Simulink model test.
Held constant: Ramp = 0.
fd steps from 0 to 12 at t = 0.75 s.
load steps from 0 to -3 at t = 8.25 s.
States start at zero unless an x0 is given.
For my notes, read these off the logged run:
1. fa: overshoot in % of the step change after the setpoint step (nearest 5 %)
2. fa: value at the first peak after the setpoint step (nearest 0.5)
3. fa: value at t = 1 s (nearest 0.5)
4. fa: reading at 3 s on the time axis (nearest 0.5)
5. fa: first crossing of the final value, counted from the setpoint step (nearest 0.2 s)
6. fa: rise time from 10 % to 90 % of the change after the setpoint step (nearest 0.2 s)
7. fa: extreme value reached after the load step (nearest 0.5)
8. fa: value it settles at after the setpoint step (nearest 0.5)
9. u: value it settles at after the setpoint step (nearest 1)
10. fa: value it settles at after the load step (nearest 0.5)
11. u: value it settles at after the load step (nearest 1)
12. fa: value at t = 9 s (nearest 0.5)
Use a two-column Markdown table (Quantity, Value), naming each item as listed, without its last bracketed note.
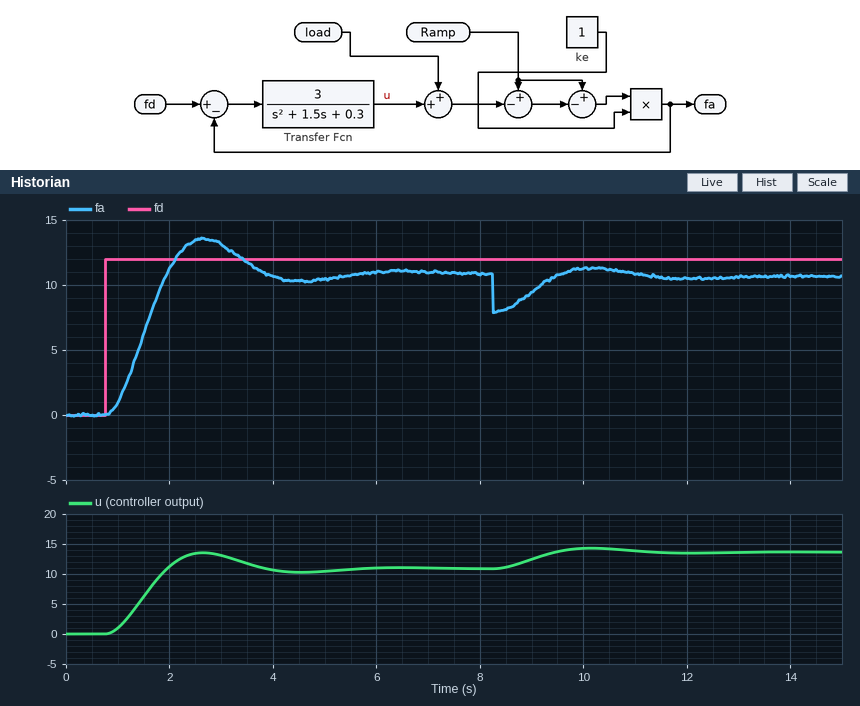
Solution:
| Quantity | Value |
|---|---|
| fa: overshoot in % of the step change after the setpoint step | 25 % |
| fa: value at the first peak after the setpoint step | 13.5 |
| fa: value at t = 1 s | 1.0 |
| fa: reading at 3 s on the time axis | 13.0 |
| fa: first crossing of the final value, counted from the setpoint step | 1.2 s |
| fa: rise time from 10 % to 90 % of the change after the setpoint step | 0.8 s |
| fa: extreme value reached after the load step | 8.0 |
| fa: value it settles at after the setpoint step | 11.0 |
| u: value it settles at after the setpoint step | 11 |
| fa: value it settles at after the load step | 10.5 |
| u: value it settles at after the load step | 14 |
| fa: value at t = 9 s | 9.5 |
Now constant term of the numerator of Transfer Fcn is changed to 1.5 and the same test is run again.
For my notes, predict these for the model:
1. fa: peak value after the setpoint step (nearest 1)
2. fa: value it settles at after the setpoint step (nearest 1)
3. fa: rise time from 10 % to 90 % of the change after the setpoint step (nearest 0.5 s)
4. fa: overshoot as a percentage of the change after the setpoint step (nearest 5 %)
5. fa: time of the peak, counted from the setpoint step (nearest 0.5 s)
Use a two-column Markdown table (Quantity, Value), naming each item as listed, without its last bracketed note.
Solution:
| Quantity | Value |
|---|---|
| fa: peak value after the setpoint step | 11 |
| fa: value it settles at after the setpoint step | 10 |
| fa: rise time from 10 % to 90 % of the change after the setpoint step | 1.5 s |
| fa: overshoot as a percentage of the change after the setpoint step | 10 % |
| fa: time of the peak, counted from the setpoint step | 3.0 s |
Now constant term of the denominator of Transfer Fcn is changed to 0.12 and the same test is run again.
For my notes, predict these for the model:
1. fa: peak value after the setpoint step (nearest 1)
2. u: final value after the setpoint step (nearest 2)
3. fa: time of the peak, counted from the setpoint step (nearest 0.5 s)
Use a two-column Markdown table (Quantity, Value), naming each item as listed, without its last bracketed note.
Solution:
| Quantity | Value |
|---|---|
| fa: peak value after the setpoint step | 14 |
| u: final value after the setpoint step | 12 |
| fa: time of the peak, counted from the setpoint step | 2.0 s |
